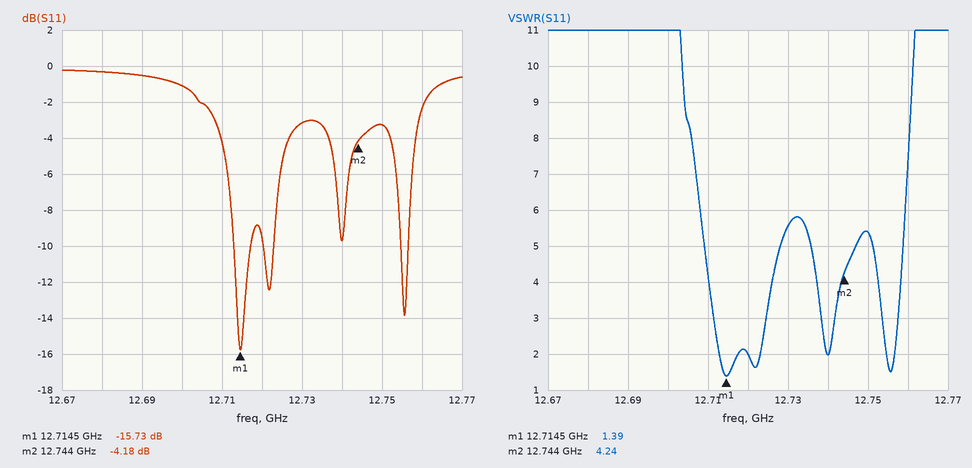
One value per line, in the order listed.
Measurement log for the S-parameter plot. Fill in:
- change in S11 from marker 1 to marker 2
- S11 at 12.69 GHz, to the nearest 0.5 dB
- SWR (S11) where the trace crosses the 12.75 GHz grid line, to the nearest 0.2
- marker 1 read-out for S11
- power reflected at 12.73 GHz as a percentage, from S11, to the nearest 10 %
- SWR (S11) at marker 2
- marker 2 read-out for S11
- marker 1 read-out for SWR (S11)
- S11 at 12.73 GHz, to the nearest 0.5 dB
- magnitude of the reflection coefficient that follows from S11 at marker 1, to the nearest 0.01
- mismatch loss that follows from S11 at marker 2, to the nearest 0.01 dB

11.55 dB
-0.5 dB
5.4
-15.73 dB
50 %
4.24
-4.18 dB
1.39
-3.0 dB
0.16
2.09 dB
